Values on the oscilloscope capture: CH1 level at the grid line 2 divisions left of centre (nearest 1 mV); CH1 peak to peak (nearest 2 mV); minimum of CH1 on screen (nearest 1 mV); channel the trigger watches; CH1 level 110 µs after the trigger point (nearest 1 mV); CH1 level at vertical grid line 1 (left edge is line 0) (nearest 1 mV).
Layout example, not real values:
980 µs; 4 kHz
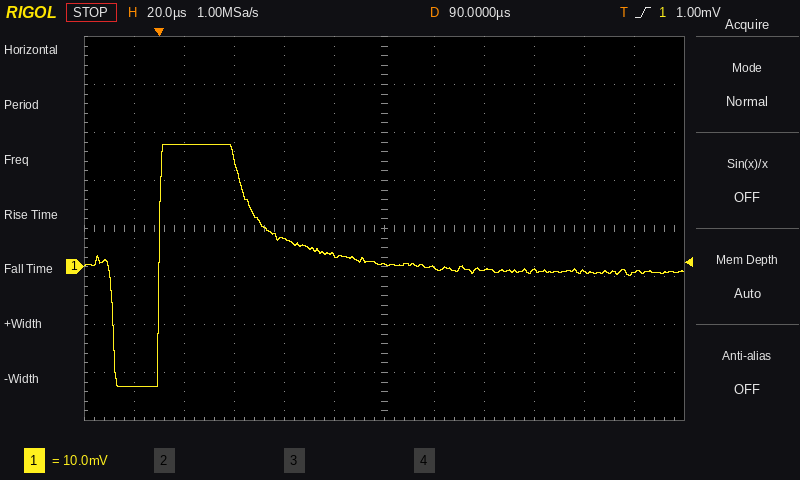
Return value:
6 mV; 50 mV; -25 mV; CH1; 0 mV; -25 mV
